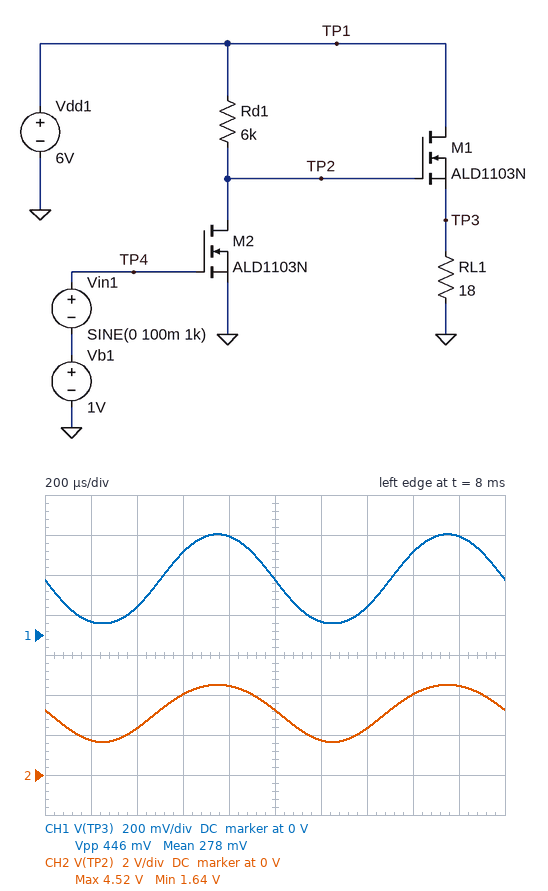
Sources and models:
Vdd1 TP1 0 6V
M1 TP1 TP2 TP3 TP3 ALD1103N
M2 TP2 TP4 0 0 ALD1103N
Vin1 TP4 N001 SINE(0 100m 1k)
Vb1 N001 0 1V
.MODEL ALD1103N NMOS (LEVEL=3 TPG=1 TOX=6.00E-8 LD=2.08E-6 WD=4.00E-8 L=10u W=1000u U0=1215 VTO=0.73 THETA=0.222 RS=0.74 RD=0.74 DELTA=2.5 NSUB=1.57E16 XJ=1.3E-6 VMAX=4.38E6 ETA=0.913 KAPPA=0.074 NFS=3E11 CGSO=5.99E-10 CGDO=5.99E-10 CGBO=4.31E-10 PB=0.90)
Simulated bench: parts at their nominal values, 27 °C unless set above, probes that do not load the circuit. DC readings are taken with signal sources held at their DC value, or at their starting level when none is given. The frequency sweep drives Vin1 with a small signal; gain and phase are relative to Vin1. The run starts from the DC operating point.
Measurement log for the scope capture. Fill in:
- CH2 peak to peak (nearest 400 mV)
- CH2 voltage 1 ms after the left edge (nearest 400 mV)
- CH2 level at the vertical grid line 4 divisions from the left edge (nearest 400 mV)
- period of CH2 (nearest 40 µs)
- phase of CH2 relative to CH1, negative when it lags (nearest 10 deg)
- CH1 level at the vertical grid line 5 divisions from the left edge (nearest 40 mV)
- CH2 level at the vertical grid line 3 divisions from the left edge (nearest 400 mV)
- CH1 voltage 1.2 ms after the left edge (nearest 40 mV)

2.8 V
3.2 V
4.4 V
1.00 ms
0 deg
280 mV
4.0 V
80 mV
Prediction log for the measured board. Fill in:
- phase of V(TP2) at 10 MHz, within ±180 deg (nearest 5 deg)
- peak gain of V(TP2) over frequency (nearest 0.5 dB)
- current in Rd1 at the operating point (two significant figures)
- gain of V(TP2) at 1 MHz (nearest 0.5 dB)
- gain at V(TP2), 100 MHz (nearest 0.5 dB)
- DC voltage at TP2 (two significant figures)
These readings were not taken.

130 deg
23.0 dB
460 µA
23.0 dB
1.5 dB
3.2 V
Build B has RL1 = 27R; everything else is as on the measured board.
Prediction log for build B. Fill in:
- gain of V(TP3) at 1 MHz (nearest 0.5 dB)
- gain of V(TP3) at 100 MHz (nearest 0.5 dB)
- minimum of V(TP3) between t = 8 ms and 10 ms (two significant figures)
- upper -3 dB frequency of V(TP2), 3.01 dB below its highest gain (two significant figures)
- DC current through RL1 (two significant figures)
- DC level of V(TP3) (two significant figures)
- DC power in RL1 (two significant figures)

10.0 dB
-11.0 dB
82 mV
8.6 MHz
14 mA
380 mV
5.4 mW
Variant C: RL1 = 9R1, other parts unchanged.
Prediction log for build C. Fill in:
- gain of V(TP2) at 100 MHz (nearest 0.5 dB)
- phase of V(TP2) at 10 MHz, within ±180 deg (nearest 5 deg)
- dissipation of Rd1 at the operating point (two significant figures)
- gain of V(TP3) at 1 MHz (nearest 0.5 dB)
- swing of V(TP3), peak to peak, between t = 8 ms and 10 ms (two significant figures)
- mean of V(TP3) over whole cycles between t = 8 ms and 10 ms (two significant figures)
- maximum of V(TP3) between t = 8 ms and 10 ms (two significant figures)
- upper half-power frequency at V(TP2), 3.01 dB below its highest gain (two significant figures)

1.0 dB
125 deg
1.3 mW
2.5 dB
250 mV
150 mV
280 mV
7.8 MHz
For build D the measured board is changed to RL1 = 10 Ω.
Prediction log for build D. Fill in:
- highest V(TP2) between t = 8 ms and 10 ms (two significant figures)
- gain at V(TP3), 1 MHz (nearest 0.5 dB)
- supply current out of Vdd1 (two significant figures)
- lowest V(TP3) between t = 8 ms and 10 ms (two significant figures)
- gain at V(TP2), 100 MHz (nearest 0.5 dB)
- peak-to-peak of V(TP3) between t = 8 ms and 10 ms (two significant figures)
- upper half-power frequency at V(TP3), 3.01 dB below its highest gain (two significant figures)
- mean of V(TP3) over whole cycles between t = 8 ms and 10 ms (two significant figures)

4.5 V
3.0 dB
17 mA
34 mV
1.0 dB
270 mV
7.8 MHz
170 mV
